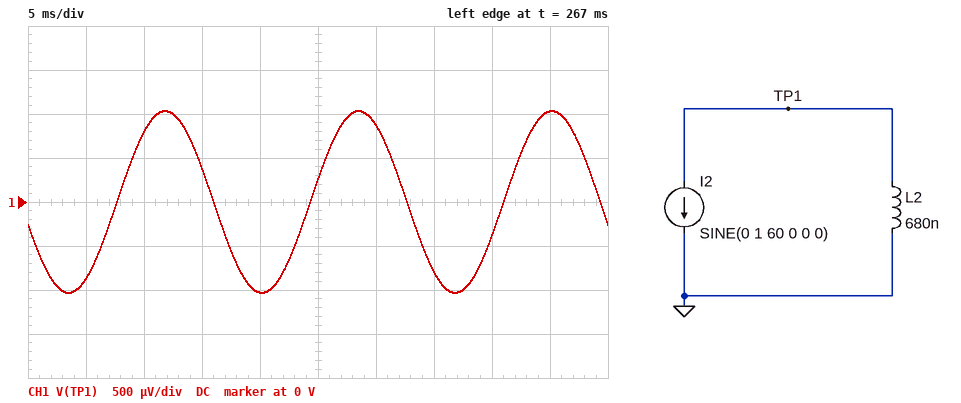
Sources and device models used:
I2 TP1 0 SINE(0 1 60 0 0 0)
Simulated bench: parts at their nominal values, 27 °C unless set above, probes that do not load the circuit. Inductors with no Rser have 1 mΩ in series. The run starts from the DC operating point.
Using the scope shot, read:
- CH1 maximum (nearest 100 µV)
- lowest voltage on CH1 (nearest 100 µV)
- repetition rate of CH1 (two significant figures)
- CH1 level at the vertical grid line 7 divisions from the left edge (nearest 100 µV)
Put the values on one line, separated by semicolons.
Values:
1.0 mV; -1.0 mV; 60 Hz; -800 µV
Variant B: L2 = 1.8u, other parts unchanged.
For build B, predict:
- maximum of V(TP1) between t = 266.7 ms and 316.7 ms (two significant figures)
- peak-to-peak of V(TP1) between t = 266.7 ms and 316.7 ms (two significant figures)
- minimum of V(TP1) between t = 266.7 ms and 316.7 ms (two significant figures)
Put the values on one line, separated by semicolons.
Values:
1.2 mV; 2.4 mV; -1.2 mV
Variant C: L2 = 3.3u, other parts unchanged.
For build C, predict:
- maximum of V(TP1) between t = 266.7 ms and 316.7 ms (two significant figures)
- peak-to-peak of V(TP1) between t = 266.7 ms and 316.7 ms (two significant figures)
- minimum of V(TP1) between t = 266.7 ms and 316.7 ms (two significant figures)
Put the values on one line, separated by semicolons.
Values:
1.6 mV; 3.2 mV; -1.6 mV
